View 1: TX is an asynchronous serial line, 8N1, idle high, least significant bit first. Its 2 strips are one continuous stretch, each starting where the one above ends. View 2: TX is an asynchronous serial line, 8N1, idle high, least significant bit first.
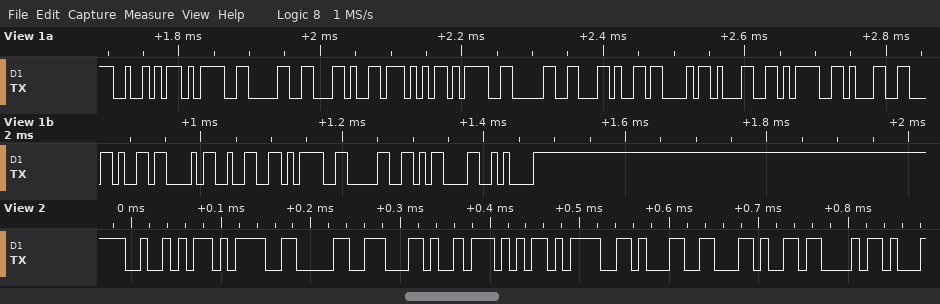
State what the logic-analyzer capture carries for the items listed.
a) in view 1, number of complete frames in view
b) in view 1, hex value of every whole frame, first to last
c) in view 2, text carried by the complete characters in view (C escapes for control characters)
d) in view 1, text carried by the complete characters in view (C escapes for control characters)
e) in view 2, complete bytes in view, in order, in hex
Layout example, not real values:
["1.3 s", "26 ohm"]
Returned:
["19", "52 3D 30 2C 57 3D 30 2C 43 31 3D 31 2C 43 32 3D 30 0D 0A", "\"R=0,W=1,C\"", "\"R=0,W=0,C1=1,C2=0\\r\\n\"", "0x52 0x3D 0x30 0x2C 0x57 0x3D 0x31 0x2C 0x43"]
